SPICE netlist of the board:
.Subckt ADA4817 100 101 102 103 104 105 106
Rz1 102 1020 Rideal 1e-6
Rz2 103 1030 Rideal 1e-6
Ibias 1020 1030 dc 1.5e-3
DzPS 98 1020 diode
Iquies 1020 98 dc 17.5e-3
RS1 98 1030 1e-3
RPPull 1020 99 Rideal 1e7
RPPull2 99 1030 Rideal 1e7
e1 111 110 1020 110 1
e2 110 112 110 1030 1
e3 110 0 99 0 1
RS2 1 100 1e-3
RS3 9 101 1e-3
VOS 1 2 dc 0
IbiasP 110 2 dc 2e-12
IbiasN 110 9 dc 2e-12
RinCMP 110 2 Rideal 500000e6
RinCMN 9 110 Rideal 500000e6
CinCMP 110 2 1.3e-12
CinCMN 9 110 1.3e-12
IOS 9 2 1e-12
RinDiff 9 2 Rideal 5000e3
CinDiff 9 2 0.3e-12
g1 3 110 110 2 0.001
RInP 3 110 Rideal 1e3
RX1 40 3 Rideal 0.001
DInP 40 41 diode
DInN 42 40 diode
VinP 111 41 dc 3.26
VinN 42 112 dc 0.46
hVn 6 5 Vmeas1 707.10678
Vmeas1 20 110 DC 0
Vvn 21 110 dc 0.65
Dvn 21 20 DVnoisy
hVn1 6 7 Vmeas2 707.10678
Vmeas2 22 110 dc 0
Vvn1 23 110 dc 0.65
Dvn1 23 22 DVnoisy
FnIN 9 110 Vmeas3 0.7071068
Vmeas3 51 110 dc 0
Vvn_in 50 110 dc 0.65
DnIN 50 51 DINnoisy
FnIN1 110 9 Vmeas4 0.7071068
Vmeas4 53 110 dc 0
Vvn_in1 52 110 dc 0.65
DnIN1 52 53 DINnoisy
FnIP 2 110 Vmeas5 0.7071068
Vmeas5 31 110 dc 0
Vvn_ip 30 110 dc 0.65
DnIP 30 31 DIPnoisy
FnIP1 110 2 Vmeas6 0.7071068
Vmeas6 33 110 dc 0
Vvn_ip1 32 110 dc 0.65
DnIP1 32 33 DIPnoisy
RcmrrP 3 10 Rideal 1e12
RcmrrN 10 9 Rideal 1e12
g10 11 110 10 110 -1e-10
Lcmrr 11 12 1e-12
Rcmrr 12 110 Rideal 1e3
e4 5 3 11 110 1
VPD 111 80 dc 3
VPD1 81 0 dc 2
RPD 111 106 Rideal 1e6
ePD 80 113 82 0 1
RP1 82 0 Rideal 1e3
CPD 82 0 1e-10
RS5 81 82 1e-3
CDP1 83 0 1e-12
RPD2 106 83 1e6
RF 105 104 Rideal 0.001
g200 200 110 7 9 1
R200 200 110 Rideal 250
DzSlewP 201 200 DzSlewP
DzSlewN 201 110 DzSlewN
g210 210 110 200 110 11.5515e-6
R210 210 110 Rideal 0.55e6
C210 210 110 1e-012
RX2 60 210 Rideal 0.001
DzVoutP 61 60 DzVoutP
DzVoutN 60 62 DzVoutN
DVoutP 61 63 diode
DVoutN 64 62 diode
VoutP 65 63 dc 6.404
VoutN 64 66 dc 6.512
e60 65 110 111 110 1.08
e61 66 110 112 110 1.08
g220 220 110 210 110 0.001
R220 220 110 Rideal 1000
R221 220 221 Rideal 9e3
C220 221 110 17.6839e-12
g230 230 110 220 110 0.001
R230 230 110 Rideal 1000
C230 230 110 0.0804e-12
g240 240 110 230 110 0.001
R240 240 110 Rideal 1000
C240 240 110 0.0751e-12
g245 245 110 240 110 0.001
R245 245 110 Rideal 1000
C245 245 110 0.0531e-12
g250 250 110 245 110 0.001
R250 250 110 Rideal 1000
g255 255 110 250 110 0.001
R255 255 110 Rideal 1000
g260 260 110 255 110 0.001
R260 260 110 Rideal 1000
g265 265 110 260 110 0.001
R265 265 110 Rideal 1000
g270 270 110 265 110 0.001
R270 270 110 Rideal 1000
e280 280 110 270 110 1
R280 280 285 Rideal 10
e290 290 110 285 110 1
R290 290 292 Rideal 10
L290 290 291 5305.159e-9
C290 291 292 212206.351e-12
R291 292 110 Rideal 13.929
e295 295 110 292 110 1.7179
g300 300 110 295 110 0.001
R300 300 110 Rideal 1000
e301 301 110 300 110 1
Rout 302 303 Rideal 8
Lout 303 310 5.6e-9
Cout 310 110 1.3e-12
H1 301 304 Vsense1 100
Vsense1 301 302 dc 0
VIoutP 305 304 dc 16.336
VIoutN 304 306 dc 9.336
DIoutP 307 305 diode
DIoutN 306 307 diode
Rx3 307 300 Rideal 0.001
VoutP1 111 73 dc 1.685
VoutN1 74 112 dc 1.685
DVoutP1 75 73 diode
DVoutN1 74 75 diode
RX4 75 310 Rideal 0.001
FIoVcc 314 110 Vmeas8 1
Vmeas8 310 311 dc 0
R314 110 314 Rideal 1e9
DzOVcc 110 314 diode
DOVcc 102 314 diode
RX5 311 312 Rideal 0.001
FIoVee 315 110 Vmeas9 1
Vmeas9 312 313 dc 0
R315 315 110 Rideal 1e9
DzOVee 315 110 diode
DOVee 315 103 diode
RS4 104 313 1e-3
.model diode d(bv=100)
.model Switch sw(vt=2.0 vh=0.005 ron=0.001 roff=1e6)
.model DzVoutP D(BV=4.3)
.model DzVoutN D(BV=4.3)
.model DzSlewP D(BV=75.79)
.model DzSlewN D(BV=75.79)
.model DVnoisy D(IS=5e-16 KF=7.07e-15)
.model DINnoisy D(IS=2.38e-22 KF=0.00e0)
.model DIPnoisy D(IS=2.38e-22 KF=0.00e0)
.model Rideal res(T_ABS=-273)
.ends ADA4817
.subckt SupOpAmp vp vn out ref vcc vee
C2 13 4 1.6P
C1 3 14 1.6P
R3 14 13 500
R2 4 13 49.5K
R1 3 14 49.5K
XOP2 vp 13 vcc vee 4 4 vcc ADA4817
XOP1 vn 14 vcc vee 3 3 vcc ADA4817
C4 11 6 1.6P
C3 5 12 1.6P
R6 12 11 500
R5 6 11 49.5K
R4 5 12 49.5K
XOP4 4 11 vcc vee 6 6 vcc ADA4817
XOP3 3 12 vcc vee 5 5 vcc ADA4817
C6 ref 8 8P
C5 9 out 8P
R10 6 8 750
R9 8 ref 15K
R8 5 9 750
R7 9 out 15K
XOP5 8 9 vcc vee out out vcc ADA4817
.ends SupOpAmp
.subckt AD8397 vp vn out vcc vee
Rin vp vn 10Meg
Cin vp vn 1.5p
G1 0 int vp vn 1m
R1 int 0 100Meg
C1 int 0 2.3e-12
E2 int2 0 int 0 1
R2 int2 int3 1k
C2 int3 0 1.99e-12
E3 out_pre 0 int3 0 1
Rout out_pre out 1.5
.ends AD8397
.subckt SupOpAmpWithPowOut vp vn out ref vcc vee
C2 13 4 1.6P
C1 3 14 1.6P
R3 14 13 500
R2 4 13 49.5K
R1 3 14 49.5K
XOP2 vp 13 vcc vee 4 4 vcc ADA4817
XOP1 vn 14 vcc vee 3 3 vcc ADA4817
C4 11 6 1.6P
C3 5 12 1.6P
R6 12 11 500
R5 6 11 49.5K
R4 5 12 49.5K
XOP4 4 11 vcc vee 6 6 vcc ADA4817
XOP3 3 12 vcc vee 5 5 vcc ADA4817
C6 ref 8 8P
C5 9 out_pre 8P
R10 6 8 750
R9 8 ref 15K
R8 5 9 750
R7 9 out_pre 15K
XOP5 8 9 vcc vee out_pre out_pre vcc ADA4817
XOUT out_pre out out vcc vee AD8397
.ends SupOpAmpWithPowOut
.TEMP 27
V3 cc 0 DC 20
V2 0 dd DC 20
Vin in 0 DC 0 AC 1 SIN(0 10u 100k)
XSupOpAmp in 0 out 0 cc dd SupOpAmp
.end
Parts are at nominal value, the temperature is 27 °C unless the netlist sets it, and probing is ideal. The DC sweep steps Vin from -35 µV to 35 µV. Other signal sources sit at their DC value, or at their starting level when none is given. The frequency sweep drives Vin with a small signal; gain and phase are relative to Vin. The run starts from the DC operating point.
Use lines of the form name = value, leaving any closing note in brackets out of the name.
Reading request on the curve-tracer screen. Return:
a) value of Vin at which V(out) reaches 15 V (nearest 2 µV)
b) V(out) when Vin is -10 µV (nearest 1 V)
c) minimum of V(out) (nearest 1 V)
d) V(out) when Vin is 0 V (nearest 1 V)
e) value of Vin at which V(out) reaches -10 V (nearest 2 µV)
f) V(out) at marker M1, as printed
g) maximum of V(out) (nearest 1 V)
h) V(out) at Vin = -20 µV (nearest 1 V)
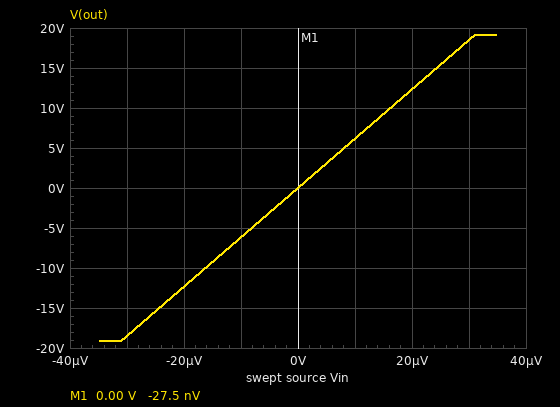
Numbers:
value of Vin at which V(out) reaches 15 V = 24 µV
V(out) when Vin is -10 µV = -6 V
minimum of V(out) = -19 V
V(out) when Vin is 0 V = 0 V
value of Vin at which V(out) reaches -10 V = -16 µV
V(out) at marker M1, as printed = -27.5 nV
maximum of V(out) = 19 V
V(out) at Vin = -20 µV = -12 V
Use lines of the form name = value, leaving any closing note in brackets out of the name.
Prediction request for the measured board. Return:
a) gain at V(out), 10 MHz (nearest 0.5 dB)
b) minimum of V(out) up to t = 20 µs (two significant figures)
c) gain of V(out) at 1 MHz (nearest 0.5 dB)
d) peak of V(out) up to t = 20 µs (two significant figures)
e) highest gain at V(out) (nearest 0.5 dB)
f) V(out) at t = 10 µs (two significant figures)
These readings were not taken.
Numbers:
gain at V(out), 10 MHz = 60.0 dB
minimum of V(out) up to t = 20 µs = -6.6 V
gain of V(out) at 1 MHz = 109.5 dB
peak of V(out) up to t = 20 µs = 6.6 V
highest gain at V(out) = 116.5 dB
V(out) at t = 10 µs = -1.2 V
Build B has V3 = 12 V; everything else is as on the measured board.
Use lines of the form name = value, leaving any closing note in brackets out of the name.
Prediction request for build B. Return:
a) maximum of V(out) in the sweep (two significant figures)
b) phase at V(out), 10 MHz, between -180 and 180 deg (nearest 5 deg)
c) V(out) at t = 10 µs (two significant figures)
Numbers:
maximum of V(out) in the sweep = 11 V
phase at V(out), 10 MHz, between -180 and 180 deg = 110 deg
V(out) at t = 10 µs = -1.3 V
